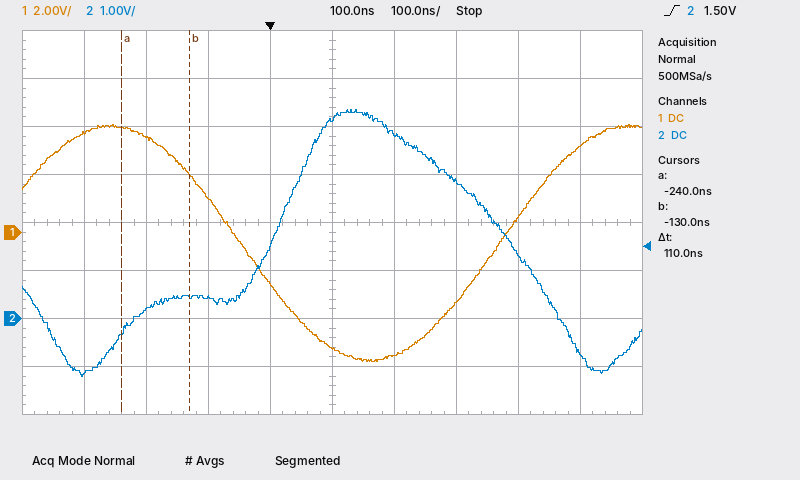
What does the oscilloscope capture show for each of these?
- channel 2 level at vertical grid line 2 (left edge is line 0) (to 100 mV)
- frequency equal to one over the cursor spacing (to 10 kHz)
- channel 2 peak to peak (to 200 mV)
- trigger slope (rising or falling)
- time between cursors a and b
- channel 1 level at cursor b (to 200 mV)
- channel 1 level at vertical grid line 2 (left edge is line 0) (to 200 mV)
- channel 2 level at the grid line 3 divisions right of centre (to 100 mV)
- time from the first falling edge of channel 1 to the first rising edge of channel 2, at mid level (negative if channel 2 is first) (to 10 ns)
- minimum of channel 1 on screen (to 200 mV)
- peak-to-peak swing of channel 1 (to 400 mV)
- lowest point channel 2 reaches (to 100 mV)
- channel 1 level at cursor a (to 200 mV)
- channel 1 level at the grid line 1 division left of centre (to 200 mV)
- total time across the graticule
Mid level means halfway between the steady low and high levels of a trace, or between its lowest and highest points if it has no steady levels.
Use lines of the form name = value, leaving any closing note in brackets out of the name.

channel 2 level at vertical grid line 2 (left edge is line 0) = 200 mV
frequency equal to one over the cursor spacing = 9.09 MHz
channel 2 peak to peak = 5.6 V
trigger slope = rising
time between cursors a and b = 110 ns
channel 1 level at cursor b = 2.4 V
channel 1 level at vertical grid line 2 (left edge is line 0) = 4.0 V
channel 2 level at the grid line 3 divisions right of centre = 1.3 V
time from the first falling edge of channel 1 to the first rising edge of channel 2, at mid level (negative if channel 2 is first) = +50 ns
minimum of channel 1 on screen = -5.4 V
peak-to-peak swing of channel 1 = 10.0 V
lowest point channel 2 reaches = -1.2 V
channel 1 level at cursor a = 4.4 V
channel 1 level at the grid line 1 division left of centre = -2.2 V
total time across the graticule = 1 µs
